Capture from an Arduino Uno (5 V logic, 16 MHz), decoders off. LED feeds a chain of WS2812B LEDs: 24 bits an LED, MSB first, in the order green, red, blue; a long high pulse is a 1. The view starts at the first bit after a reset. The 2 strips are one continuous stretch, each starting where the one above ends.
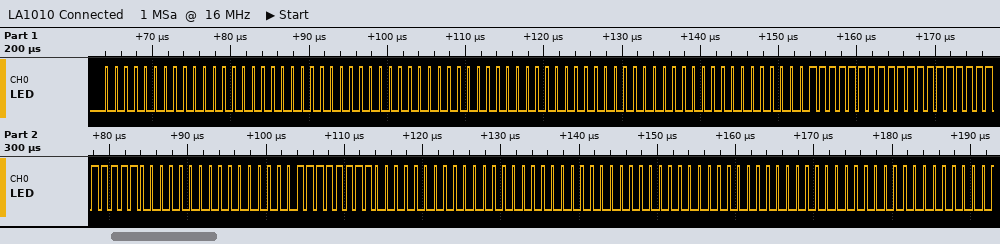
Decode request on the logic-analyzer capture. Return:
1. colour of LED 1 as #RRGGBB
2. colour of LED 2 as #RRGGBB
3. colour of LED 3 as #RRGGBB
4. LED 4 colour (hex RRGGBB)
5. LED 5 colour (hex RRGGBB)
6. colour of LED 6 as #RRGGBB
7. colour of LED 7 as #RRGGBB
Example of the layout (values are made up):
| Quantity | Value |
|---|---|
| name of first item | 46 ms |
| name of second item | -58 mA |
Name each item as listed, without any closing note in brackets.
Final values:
| Quantity | Value |
|---|---|
| colour of LED 1 as #RRGGBB | #000000 |
| colour of LED 2 as #RRGGBB | #000000 |
| colour of LED 3 as #RRGGBB | #000000 |
| LED 4 colour | #FFFFFF |
| LED 5 colour | #0000FF |
| colour of LED 6 as #RRGGBB | #000000 |
| colour of LED 7 as #RRGGBB | #000000 |
